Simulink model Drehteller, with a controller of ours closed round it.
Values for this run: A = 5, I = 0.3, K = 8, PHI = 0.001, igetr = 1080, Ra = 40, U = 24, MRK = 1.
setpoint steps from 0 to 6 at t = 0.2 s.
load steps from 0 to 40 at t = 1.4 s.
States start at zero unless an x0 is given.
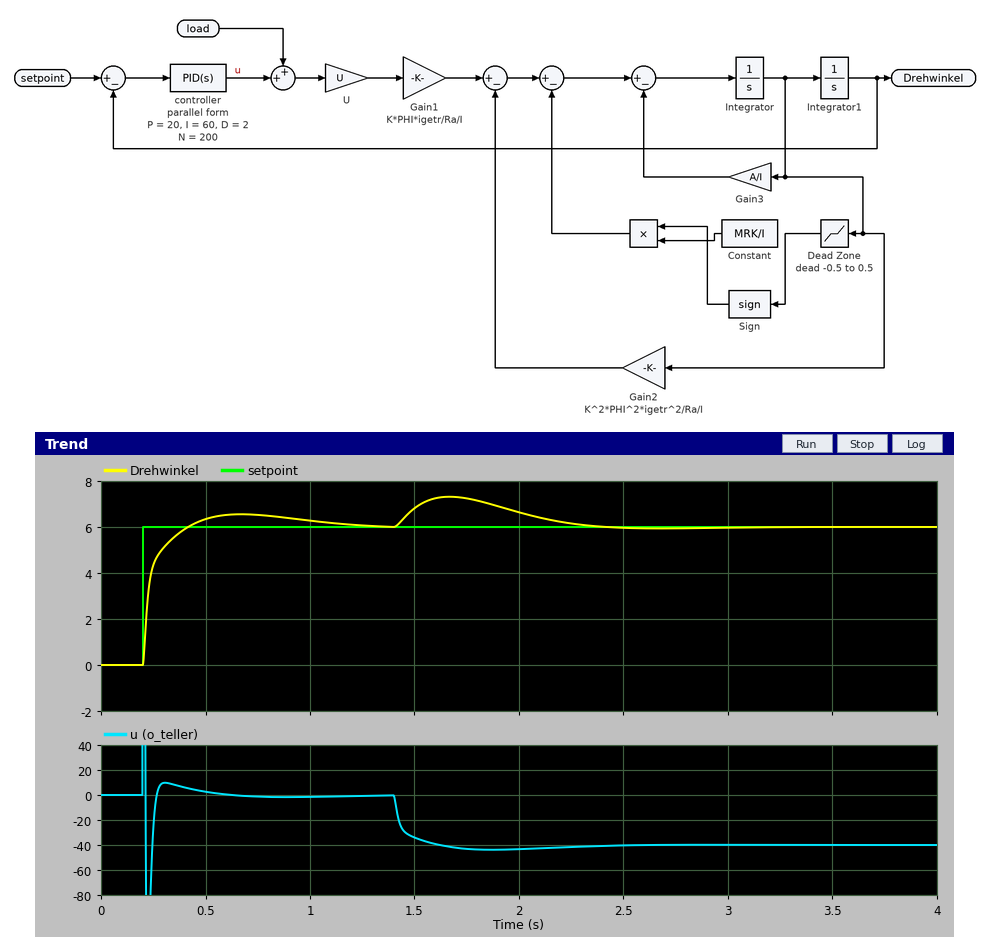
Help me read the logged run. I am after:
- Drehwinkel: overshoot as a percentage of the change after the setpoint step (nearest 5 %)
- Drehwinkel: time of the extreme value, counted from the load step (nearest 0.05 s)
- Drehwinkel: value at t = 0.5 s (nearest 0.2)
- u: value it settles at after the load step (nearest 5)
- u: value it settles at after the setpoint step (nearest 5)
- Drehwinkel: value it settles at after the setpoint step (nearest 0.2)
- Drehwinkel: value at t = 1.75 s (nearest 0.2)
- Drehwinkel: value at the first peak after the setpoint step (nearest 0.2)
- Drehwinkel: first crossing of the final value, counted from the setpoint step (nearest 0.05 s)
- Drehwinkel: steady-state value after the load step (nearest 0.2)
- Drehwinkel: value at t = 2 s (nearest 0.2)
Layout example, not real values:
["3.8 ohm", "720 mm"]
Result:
["10 %", "0.25 s", "6.4", "-40", "0", "6.0", "7.2", "6.6", "0.20 s", "6.0", "6.6"]
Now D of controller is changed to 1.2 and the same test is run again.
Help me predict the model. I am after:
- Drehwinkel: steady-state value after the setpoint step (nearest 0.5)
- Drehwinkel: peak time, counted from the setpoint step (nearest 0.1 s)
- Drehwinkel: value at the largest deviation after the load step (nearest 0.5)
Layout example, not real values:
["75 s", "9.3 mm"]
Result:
["6.0", "0.4 s", "7.5"]
